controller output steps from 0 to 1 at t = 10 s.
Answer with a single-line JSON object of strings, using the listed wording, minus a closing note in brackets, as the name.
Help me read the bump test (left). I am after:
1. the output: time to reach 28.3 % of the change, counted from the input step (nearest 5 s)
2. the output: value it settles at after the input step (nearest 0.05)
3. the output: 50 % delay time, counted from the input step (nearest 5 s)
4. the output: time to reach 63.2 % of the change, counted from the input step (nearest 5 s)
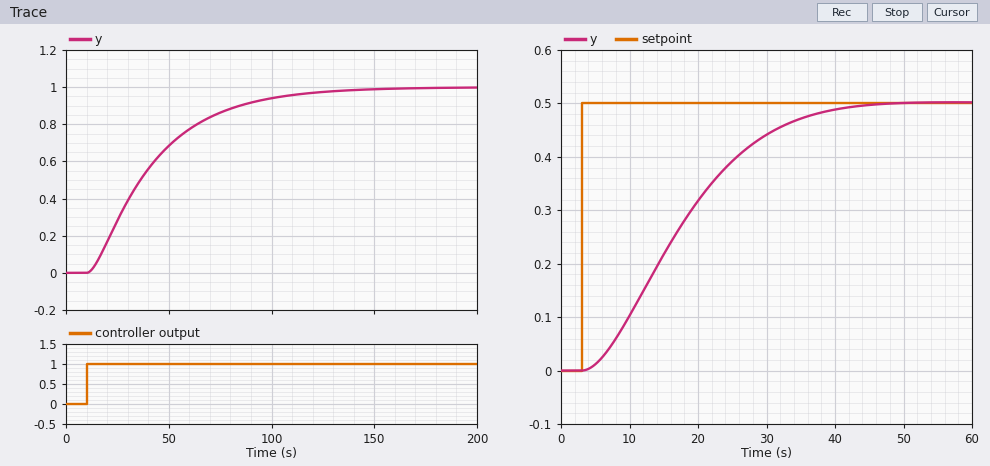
{"the output: time to reach 28.3 % of the change, counted from the input step": "15 s", "the output: value it settles at after the input step": "1.00", "the output: 50 % delay time, counted from the input step": "25 s", "the output: time to reach 63.2 % of the change, counted from the input step": "35 s"}
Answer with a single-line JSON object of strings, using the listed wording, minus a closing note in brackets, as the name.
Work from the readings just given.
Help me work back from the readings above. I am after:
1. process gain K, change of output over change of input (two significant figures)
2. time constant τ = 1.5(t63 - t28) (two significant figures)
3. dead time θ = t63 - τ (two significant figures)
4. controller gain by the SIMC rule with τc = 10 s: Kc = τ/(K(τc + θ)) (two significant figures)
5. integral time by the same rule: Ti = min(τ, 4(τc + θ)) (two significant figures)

{"process gain K, change of output over change of input": "1.0", "time constant τ = 1.5(t63 - t28)": "30 s", "dead time θ = t63 - τ": "5.0 s", "controller gain by the SIMC rule with τc = 10 s: Kc = τ/(K(τc + θ))": "2.0", "integral time by the same rule: Ti = min(τ, 4(τc + θ))": "30 s"}
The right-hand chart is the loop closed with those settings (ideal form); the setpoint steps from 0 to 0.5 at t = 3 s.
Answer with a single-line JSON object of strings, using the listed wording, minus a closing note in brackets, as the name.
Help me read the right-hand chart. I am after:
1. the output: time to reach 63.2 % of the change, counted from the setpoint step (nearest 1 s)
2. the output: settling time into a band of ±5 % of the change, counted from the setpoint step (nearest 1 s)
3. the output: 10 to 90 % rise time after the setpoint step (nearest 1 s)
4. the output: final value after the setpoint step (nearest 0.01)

{"the output: time to reach 63.2 % of the change, counted from the setpoint step": "17 s", "the output: settling time into a band of ±5 % of the change, counted from the setpoint step": "33 s", "the output: 10 to 90 % rise time after the setpoint step": "24 s", "the output: final value after the setpoint step": "0.50"}
